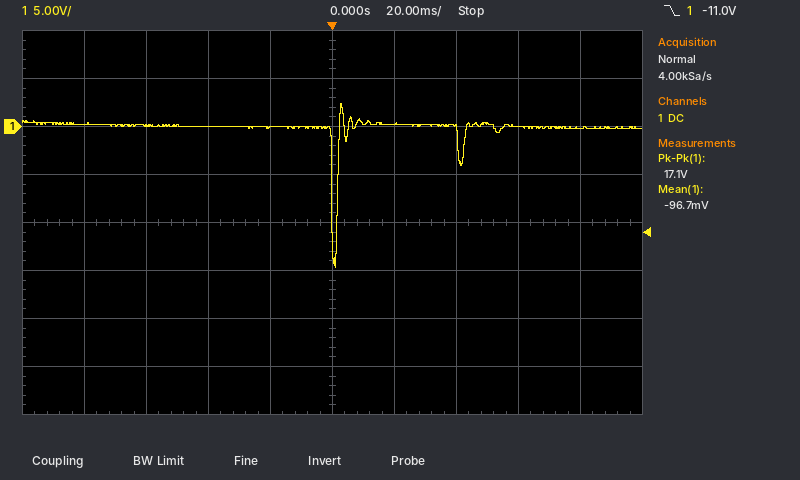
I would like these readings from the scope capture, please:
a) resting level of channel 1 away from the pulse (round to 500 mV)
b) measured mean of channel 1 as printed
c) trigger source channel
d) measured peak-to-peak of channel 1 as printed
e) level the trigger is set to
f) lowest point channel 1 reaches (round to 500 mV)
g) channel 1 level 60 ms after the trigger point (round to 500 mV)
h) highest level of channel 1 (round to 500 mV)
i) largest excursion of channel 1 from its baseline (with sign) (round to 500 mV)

0.0 V
-96.7 mV
channel 1
17.1 V
-11.0 V
-14.5 V
0.0 V
2.5 V
-14.5 V
